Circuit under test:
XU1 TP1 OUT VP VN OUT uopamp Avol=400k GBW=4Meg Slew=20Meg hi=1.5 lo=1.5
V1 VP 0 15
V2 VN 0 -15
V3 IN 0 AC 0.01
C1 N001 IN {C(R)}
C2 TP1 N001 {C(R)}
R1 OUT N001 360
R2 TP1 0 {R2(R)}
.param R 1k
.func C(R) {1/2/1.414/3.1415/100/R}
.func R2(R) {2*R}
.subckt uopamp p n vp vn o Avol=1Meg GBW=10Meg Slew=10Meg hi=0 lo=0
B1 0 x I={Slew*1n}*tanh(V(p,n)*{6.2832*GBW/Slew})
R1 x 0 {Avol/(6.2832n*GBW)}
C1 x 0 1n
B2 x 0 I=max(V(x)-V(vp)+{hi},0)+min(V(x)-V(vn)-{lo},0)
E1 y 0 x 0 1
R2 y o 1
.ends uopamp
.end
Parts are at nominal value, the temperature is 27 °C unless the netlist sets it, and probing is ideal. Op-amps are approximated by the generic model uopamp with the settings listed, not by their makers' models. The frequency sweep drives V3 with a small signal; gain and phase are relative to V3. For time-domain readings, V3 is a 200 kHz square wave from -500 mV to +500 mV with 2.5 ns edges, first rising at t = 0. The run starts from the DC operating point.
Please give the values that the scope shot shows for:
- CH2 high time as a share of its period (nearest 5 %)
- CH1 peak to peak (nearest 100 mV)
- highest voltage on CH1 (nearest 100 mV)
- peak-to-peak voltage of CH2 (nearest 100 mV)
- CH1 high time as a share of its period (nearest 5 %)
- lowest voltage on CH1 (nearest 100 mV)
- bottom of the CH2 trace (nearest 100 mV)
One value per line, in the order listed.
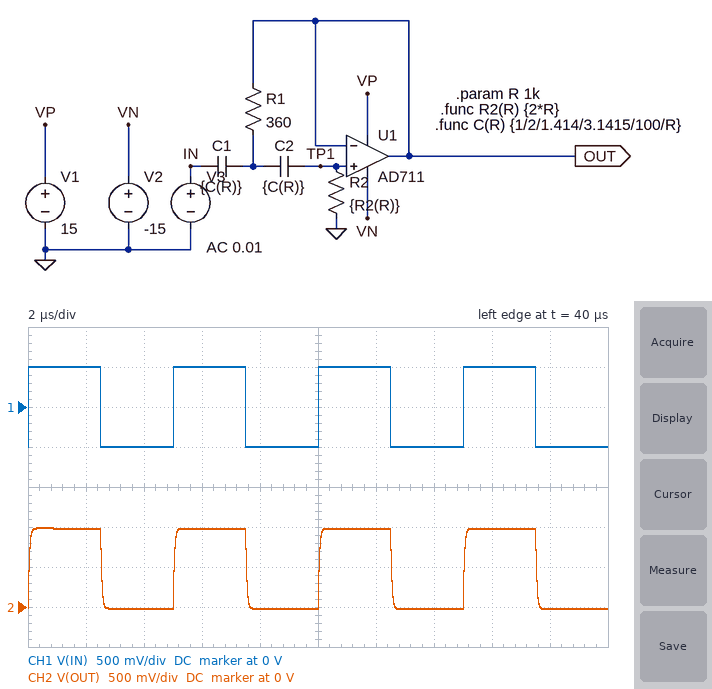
50 %
1.0 V
500 mV
1.0 V
50 %
-500 mV
0 V
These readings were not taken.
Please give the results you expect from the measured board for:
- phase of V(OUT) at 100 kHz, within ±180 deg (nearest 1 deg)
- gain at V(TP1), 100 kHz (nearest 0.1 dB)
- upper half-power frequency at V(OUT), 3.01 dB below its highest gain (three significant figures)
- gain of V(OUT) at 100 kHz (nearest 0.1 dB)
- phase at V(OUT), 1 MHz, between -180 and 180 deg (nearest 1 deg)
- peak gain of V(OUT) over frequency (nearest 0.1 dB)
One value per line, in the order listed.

-1 deg
0 dB
1.70 MHz
0 dB
-14 deg
2.3 dB
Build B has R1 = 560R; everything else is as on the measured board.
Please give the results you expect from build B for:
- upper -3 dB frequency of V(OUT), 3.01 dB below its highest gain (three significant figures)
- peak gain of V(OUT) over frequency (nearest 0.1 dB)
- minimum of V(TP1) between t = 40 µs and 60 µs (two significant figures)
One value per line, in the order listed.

3.13 MHz
0.9 dB
-27 mV
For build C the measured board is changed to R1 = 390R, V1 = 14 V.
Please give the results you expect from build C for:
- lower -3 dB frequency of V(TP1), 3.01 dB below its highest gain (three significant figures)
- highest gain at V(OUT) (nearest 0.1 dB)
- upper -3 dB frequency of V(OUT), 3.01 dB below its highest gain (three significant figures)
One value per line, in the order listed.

135 Hz
2.0 dB
2.02 MHz
